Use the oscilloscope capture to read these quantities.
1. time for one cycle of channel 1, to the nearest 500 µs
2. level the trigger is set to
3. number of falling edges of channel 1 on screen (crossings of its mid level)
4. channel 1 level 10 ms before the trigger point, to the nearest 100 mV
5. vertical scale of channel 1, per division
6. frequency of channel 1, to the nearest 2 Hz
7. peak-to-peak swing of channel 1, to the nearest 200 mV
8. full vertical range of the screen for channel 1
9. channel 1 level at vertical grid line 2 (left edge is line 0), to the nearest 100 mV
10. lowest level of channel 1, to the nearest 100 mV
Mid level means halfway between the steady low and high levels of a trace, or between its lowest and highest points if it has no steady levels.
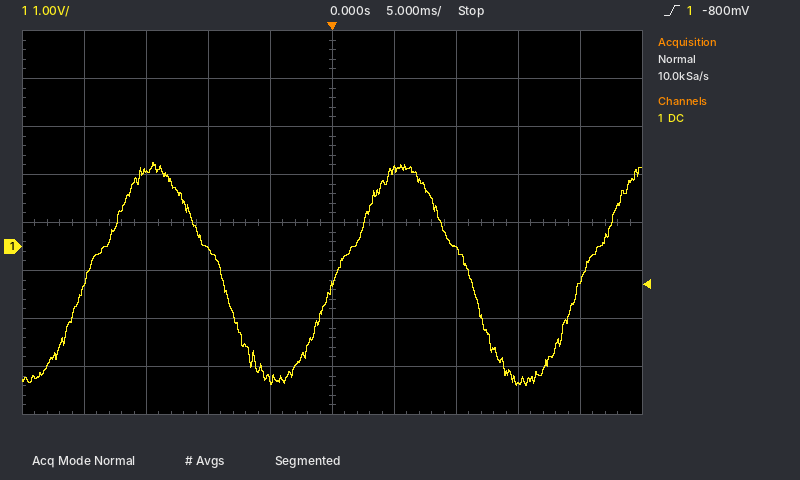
20.0 ms
-800 mV
2
-100 mV
1 V
50 Hz
4.6 V
8 V
1.6 V
-2.9 V
